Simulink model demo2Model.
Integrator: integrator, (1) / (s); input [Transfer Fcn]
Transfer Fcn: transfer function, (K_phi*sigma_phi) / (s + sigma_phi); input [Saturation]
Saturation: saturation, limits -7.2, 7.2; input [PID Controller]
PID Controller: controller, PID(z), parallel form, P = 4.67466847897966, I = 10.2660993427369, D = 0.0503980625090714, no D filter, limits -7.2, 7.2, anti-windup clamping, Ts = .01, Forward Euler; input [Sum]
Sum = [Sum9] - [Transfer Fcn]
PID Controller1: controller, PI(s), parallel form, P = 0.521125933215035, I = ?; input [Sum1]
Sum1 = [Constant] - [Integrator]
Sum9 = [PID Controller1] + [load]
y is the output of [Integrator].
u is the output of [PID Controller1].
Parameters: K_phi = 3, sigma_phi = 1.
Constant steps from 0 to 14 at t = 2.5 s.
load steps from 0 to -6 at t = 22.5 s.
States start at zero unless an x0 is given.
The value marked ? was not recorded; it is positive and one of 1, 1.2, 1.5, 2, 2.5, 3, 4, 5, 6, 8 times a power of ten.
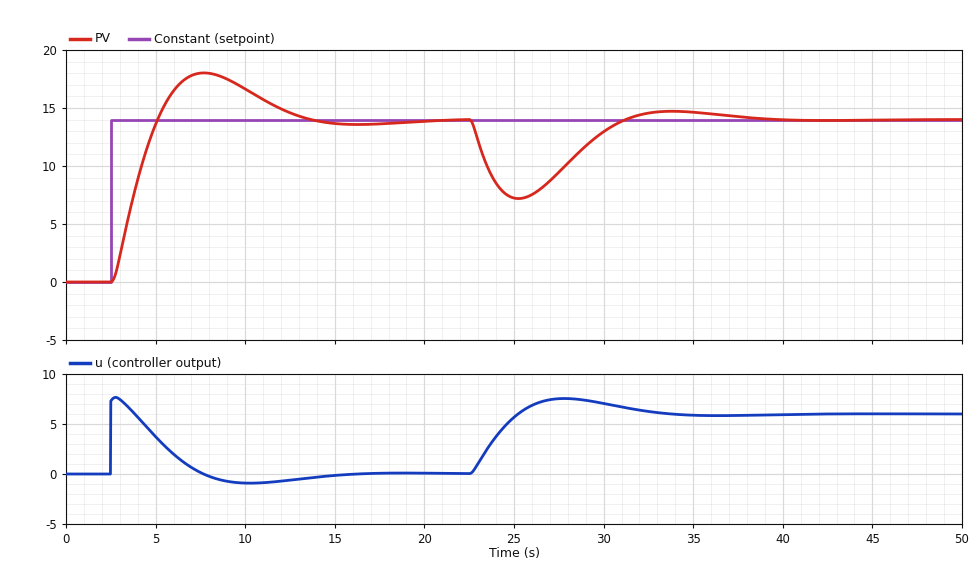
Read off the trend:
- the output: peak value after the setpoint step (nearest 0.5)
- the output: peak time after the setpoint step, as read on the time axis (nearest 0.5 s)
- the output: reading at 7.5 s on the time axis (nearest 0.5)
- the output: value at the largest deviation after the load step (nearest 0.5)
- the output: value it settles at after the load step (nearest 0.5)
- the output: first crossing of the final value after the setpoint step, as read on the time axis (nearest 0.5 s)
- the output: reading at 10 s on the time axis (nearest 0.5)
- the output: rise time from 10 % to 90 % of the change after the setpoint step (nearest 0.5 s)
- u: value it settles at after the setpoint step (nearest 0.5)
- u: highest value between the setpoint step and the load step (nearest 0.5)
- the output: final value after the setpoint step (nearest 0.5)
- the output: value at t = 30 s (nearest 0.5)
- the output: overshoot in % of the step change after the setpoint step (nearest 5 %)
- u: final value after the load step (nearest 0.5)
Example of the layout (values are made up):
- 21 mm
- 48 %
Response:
- 18.0
- 7.5 s
- 18.0
- 7.0
- 14.0
- 5.0 s
- 16.5
- 2.0 s
- 0.0
- 7.5
- 14.0
- 13.0
- 30 %
- 6.0
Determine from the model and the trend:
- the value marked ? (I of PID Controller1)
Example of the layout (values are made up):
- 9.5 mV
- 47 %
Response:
- 0.2
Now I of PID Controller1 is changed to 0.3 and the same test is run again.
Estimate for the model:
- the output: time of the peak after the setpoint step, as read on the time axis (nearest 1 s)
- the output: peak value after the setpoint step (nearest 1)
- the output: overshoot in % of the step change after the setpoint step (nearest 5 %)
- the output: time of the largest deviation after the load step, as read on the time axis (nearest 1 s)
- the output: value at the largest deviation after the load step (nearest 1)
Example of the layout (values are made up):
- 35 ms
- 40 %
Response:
- 7 s
- 19
- 35 %
- 25 s
- 8
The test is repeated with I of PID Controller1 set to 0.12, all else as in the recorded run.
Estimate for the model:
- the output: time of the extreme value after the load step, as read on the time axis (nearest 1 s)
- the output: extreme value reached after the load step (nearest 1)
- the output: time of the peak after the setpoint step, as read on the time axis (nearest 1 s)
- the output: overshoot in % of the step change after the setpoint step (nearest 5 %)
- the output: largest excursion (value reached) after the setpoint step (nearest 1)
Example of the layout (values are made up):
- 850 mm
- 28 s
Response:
- 26 s
- 6
- 9 s
- 20 %
- 17
